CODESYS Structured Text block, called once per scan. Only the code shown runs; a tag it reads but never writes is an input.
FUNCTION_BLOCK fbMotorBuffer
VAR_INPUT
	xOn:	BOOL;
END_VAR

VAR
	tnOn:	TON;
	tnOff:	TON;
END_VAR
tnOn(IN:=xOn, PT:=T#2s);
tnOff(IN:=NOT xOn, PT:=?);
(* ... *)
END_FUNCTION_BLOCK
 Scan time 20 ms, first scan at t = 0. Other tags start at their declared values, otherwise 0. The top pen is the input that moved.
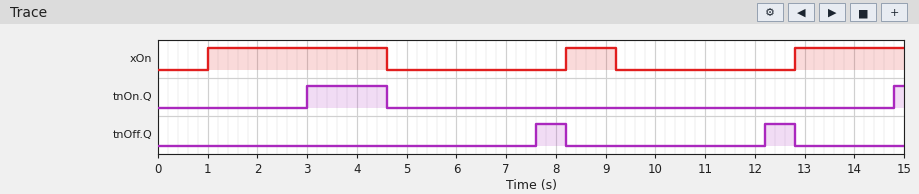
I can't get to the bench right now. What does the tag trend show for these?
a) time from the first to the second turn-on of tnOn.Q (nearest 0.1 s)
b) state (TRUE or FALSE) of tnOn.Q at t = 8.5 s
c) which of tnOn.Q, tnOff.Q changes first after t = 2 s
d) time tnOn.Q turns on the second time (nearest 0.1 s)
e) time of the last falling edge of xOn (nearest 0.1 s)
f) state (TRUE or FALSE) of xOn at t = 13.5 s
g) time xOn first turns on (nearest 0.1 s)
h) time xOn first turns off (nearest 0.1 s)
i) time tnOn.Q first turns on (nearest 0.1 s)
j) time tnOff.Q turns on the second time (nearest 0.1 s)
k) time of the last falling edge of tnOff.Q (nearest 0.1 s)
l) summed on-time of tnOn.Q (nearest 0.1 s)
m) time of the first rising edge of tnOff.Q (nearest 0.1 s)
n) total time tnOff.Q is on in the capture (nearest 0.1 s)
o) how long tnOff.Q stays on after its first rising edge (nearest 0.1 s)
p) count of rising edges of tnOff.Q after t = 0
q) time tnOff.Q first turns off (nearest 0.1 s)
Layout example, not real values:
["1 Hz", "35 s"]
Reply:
["11.8 s", "FALSE", "tnOn.Q", "14.8 s", "9.2 s", "TRUE", "1.0 s", "4.6 s", "3.0 s", "12.2 s", "12.8 s", "1.8 s", "7.6 s", "1.2 s", "0.6 s", "2", "8.2 s"]
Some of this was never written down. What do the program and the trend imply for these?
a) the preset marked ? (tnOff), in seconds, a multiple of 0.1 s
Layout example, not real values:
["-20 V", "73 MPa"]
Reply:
["3.0 s"]
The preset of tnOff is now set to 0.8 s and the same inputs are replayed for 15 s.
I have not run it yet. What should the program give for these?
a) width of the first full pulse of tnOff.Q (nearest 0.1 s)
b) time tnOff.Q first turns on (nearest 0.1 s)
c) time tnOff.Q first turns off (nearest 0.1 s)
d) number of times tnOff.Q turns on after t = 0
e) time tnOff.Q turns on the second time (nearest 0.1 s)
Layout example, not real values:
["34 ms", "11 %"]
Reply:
["0.2 s", "0.8 s", "1.0 s", "3", "5.4 s"]
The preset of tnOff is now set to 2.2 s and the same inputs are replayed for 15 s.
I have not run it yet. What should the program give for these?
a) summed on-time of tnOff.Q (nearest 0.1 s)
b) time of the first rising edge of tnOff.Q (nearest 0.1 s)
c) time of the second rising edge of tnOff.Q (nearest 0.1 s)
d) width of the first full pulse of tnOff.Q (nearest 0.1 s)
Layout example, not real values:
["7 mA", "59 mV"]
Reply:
["2.8 s", "6.8 s", "11.4 s", "1.4 s"]
